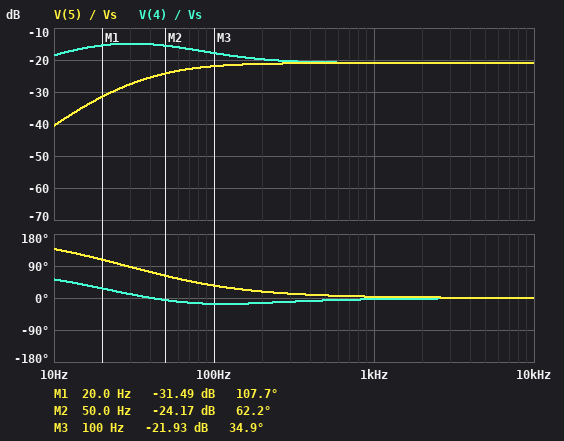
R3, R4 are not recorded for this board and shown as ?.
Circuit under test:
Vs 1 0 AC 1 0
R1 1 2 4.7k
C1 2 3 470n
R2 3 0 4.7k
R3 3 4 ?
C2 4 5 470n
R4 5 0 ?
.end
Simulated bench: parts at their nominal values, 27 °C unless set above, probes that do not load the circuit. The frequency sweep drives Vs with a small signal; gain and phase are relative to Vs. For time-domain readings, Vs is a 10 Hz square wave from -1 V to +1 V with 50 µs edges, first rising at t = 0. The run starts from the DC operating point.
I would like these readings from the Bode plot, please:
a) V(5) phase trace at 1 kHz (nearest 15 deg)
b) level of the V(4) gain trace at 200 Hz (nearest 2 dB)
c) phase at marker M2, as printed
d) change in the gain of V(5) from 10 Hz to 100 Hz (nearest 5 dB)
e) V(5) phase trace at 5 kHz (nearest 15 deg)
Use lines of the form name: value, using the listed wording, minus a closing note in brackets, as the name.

V(5) phase trace at 1 kHz: 0 deg
level of the V(4) gain trace at 200 Hz: -20 dB
phase at marker M2, as printed: 62.2 deg
change in the gain of V(5) from 10 Hz to 100 Hz: 20 dB
V(5) phase trace at 5 kHz: 0 deg
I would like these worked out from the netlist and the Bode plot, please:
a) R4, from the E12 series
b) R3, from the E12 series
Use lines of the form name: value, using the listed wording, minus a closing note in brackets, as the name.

R4, from the E12 series: 2.7 kΩ
R3, from the E12 series: 10 kΩ
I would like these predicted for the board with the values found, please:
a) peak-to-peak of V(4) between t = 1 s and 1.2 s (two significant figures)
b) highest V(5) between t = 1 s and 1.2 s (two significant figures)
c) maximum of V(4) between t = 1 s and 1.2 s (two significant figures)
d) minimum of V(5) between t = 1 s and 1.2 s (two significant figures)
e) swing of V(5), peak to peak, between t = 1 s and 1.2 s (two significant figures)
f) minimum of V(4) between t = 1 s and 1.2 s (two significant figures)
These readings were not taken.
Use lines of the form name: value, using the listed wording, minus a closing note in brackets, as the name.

peak-to-peak of V(4) between t = 1 s and 1.2 s: 550 mV
highest V(5) between t = 1 s and 1.2 s: 180 mV
maximum of V(4) between t = 1 s and 1.2 s: 280 mV
minimum of V(5) between t = 1 s and 1.2 s: -180 mV
swing of V(5), peak to peak, between t = 1 s and 1.2 s: 360 mV
minimum of V(4) between t = 1 s and 1.2 s: -280 mV
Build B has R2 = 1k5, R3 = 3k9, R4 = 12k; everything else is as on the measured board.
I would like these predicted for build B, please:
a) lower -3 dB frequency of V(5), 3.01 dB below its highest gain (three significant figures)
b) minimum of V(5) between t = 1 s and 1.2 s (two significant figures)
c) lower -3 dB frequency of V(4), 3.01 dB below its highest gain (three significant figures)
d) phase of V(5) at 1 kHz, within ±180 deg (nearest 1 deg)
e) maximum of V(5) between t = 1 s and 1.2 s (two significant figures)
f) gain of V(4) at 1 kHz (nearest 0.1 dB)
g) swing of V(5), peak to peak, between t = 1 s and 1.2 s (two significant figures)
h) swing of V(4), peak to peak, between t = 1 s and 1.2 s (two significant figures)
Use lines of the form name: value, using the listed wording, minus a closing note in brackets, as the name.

lower -3 dB frequency of V(5), 3.01 dB below its highest gain: 62.1 Hz
minimum of V(5) between t = 1 s and 1.2 s: -340 mV
lower -3 dB frequency of V(4), 3.01 dB below its highest gain: 49.4 Hz
phase of V(5) at 1 kHz, within ±180 deg: 4 deg
maximum of V(5) between t = 1 s and 1.2 s: 340 mV
gain of V(4) at 1 kHz: -15.4 dB
swing of V(5), peak to peak, between t = 1 s and 1.2 s: 670 mV
swing of V(4), peak to peak, between t = 1 s and 1.2 s: 680 mV
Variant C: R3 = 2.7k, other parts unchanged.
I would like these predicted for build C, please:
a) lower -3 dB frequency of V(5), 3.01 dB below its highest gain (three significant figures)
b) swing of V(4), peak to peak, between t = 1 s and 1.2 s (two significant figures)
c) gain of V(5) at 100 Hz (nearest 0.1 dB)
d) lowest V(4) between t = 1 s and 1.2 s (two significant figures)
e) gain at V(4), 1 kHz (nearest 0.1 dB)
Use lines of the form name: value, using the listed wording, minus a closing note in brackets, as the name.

lower -3 dB frequency of V(5), 3.01 dB below its highest gain: 74.3 Hz
swing of V(4), peak to peak, between t = 1 s and 1.2 s: 810 mV
gain of V(5) at 100 Hz: -17.0 dB
lowest V(4) between t = 1 s and 1.2 s: -410 mV
gain at V(4), 1 kHz: -15.1 dB
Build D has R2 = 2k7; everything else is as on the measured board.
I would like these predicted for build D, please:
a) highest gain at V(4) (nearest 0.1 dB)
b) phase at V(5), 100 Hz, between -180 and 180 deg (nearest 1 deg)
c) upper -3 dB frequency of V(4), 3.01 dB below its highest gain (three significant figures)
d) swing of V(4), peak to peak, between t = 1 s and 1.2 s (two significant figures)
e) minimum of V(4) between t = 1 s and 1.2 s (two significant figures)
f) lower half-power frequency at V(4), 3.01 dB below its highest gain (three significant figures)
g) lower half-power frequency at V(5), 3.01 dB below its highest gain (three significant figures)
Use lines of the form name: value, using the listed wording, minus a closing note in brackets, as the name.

highest gain at V(4): -18.2 dB
phase at V(5), 100 Hz, between -180 and 180 deg: 39 deg
upper -3 dB frequency of V(4), 3.01 dB below its highest gain: 132 Hz
swing of V(4), peak to peak, between t = 1 s and 1.2 s: 380 mV
minimum of V(4) between t = 1 s and 1.2 s: -190 mV
lower half-power frequency at V(4), 3.01 dB below its highest gain: 13.2 Hz
lower half-power frequency at V(5), 3.01 dB below its highest gain: 58.5 Hz
